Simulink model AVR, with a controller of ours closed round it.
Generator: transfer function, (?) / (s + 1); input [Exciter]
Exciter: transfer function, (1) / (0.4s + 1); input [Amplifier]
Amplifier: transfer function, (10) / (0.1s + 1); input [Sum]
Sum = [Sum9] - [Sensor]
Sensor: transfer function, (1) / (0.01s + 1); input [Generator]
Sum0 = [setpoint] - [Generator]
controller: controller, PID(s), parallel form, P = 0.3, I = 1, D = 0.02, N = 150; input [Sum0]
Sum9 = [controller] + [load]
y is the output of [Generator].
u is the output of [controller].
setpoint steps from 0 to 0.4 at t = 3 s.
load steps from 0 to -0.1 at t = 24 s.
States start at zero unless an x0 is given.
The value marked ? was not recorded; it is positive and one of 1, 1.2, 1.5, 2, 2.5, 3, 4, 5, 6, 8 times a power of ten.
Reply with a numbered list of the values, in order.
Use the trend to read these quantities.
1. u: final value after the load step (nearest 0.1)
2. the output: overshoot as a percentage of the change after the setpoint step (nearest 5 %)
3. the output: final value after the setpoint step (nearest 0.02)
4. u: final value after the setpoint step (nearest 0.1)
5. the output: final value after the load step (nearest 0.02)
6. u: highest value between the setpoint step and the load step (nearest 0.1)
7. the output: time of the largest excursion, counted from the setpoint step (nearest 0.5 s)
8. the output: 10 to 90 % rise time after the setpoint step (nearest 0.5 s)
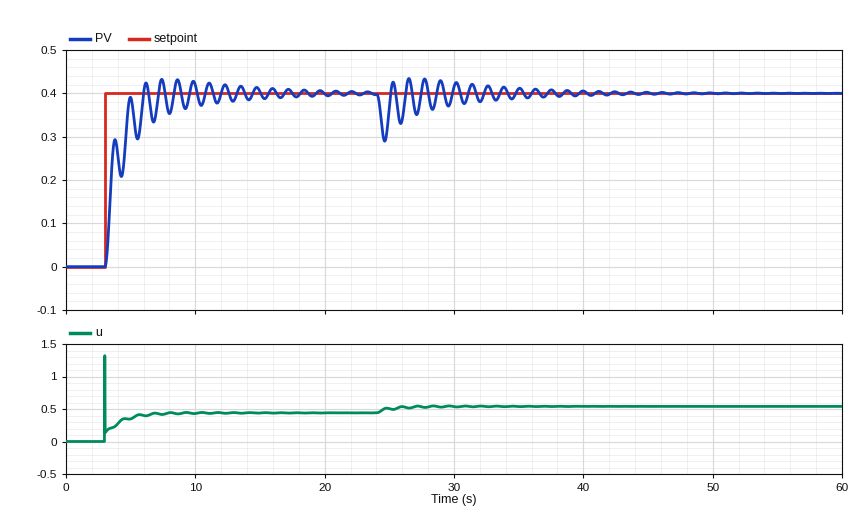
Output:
1. 0.5
2. 10 %
3. 0.40
4. 0.4
5. 0.40
6. 1.3
7. 4.5 s
8. 1.5 s
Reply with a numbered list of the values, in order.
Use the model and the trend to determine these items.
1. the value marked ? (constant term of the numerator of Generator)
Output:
1. 1
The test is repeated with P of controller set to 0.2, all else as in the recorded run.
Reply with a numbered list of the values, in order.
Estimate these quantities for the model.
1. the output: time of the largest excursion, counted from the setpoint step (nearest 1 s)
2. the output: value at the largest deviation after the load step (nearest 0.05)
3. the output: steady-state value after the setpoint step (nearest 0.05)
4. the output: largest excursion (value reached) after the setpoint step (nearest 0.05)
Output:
1. 5 s
2. 0.30
3. 0.40
4. 0.40
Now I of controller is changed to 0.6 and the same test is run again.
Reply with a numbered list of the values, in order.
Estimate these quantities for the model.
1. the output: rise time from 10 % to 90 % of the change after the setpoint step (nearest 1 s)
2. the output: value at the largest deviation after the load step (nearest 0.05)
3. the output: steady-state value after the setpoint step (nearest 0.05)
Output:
1. 4 s
2. 0.30
3. 0.40
